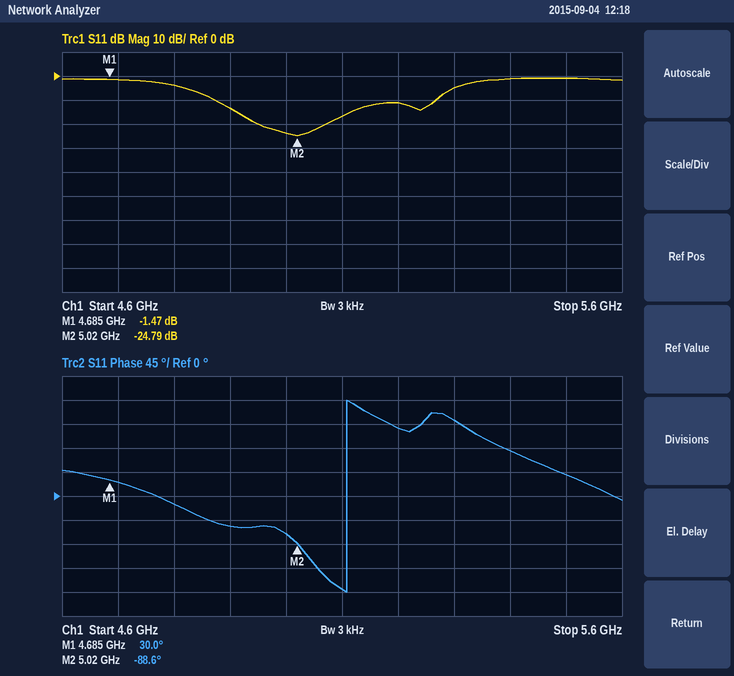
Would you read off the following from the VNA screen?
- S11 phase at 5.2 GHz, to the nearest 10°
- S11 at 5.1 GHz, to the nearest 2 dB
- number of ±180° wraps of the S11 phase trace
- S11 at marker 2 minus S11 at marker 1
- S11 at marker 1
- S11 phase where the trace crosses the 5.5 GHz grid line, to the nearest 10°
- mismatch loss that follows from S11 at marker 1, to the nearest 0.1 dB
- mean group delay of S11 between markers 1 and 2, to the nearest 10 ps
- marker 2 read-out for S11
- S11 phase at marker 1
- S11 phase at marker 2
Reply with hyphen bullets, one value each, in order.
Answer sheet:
- 130°
- -16 dB
- 1
- -23.32 dB
- -1.47 dB
- 40°
- 5.4 dB
- 980 ps
- -24.79 dB
- 30.0°
- -88.6°
